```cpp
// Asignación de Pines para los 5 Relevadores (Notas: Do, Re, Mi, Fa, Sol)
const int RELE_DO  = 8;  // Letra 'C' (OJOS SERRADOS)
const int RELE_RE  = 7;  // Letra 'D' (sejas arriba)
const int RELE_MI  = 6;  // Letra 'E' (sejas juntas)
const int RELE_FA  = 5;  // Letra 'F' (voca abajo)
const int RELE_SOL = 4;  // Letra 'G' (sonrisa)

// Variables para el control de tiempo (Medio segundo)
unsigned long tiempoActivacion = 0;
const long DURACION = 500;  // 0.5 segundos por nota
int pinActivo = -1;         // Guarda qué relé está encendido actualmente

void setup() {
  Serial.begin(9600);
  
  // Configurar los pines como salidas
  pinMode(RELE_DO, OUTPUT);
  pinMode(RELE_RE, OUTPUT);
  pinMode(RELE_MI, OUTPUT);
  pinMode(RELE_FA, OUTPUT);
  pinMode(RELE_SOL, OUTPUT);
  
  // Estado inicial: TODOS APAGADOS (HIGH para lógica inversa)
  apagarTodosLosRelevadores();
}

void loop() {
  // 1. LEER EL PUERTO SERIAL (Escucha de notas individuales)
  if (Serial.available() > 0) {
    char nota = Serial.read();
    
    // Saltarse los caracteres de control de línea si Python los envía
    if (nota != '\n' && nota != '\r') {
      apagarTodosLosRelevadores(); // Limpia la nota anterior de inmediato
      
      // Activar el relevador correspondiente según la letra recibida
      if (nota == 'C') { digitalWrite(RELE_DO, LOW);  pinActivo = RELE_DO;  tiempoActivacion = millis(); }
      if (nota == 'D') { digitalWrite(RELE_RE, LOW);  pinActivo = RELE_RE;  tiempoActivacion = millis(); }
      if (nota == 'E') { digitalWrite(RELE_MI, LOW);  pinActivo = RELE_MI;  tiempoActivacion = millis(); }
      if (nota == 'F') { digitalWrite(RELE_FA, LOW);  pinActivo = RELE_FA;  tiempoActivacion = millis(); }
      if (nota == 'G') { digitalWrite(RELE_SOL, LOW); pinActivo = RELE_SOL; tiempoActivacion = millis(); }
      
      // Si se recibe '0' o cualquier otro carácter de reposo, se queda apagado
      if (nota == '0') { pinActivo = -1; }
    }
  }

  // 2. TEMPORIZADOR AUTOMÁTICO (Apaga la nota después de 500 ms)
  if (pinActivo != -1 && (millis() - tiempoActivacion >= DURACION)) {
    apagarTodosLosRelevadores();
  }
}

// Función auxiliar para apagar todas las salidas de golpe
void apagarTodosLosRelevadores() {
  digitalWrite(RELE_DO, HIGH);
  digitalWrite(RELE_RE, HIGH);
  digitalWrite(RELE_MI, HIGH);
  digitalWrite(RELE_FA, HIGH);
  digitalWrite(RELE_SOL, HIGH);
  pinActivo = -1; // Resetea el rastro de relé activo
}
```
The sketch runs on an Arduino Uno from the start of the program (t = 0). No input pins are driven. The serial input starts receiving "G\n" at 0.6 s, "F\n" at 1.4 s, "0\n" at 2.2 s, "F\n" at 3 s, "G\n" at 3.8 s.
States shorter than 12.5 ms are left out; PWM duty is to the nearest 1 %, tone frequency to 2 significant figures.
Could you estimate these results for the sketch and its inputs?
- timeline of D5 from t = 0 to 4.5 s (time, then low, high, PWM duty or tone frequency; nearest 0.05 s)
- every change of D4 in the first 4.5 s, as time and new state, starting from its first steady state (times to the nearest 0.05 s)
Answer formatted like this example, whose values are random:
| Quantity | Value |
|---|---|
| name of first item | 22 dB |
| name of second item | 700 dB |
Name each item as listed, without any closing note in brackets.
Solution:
| Quantity | Value |
|---|---|
| timeline of D5 from t = 0 to 4.5 s | 0 s high; 1.4 s low; 1.9 s high; 3 s low; 3.5 s high |
| every change of D4 in the first 4.5 s, as time and new state, starting from its first steady state | 0 s high; 0.6 s low; 1.1 s high; 3.8 s low; 4.3 s high |
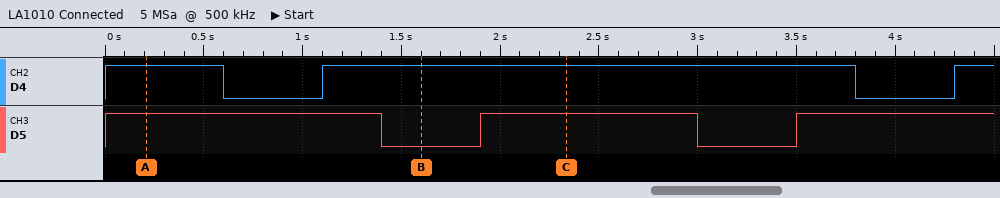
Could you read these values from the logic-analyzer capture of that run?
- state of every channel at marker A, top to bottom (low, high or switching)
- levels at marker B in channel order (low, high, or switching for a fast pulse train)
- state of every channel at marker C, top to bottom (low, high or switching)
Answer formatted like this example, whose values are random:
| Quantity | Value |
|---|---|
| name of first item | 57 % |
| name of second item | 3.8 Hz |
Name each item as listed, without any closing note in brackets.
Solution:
| Quantity | Value |
|---|---|
| state of every channel at marker A, top to bottom | D4 high, D5 high |
| levels at marker B in channel order | D4 high, D5 low |
| state of every channel at marker C, top to bottom | D4 high, D5 high |
